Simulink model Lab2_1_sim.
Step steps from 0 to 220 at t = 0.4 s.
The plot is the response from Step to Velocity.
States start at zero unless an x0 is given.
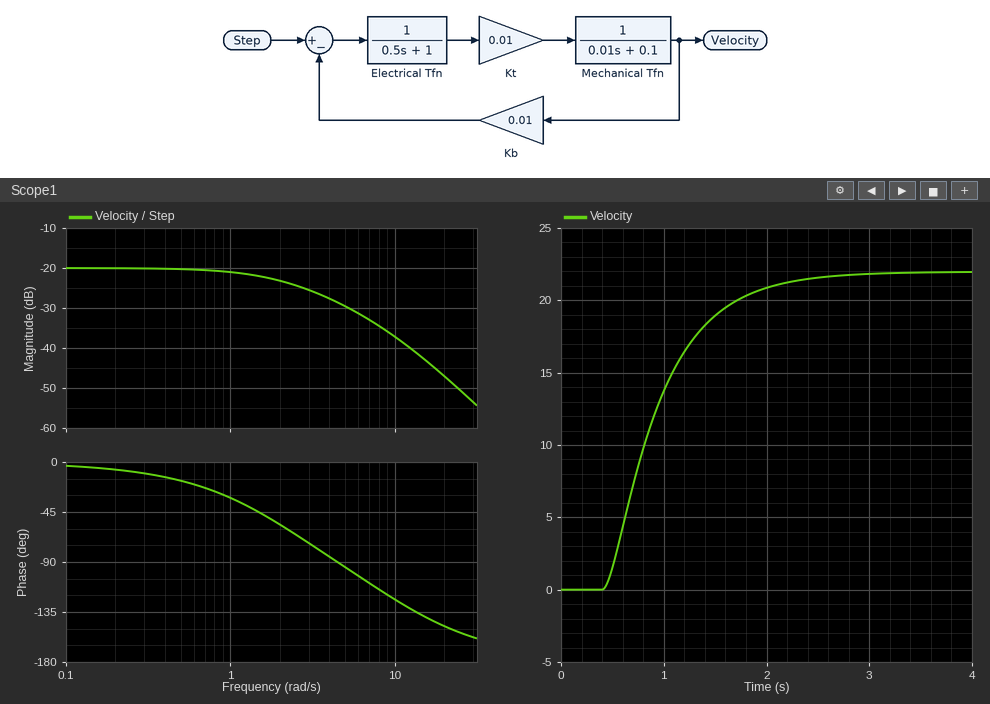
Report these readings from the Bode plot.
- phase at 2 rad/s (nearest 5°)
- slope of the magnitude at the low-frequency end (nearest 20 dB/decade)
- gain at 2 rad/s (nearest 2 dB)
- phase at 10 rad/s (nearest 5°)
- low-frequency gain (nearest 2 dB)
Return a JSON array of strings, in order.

["-55°", "0 dB/decade", "-24 dB", "-125°", "-20 dB"]
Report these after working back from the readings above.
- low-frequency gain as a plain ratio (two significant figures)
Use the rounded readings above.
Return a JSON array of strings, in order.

["0.10"]
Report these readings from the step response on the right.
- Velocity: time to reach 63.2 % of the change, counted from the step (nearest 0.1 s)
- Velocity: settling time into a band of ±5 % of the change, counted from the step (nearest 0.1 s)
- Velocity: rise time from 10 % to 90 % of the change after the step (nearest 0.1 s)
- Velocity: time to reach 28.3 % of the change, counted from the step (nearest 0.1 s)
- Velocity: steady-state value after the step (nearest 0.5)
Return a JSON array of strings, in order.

["0.6 s", "1.6 s", "1.1 s", "0.3 s", "22.0"]
